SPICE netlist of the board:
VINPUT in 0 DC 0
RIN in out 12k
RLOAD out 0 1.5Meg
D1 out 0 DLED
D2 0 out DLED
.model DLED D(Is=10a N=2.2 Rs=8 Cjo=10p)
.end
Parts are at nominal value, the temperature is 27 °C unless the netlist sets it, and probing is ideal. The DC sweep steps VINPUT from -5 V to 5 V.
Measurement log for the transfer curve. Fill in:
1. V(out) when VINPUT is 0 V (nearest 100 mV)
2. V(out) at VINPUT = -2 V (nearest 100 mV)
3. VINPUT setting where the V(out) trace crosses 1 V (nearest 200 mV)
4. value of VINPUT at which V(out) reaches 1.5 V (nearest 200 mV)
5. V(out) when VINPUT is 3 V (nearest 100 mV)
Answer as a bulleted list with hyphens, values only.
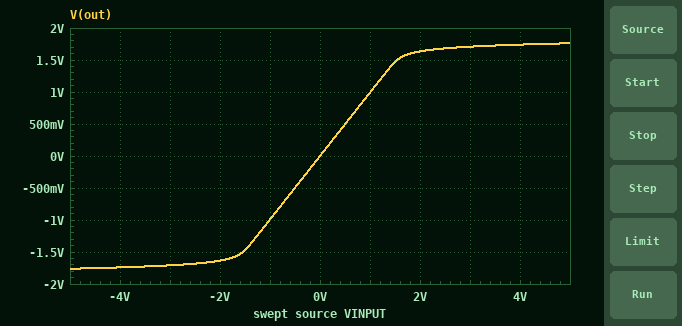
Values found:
- 0 V
- -1.6 V
- 1.0 V
- 1.6 V
- 1.7 V
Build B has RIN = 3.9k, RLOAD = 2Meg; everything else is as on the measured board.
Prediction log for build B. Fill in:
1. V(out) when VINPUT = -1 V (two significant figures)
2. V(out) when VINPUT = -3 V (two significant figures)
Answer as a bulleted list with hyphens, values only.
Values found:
- -1.0 V
- -1.8 V
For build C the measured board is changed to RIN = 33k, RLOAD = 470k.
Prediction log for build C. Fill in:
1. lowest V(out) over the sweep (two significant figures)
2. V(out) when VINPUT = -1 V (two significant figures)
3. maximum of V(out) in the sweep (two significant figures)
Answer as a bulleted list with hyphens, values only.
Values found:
- -1.7 V
- -930 mV
- 1.7 V
